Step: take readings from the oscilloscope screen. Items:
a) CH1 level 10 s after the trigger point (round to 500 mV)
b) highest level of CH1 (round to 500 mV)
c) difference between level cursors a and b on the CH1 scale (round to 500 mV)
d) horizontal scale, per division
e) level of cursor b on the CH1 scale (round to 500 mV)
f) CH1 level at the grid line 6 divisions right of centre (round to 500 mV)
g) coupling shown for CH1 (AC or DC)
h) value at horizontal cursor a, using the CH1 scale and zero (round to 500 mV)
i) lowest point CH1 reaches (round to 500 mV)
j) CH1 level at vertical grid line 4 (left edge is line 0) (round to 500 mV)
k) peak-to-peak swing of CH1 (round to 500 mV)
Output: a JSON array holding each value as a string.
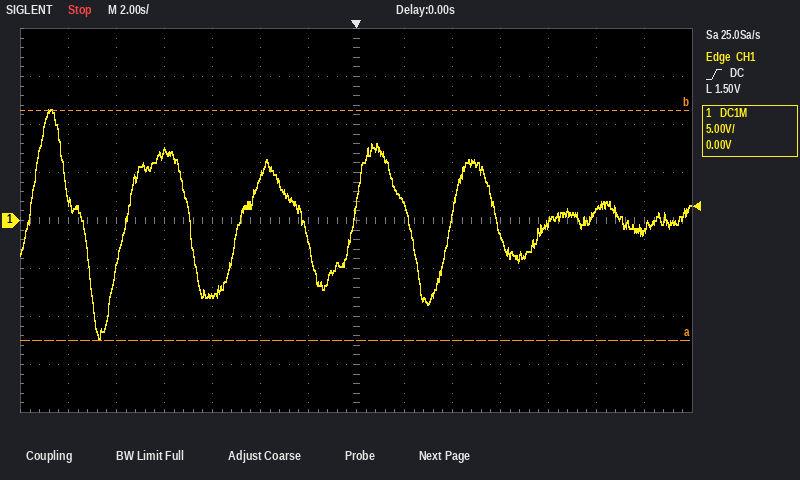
["1.0 V", "11.5 V", "24.0 V", "2 s", "11.5 V", "-1.0 V", "DC", "-12.5 V", "-12.5 V", "-8.0 V", "24.0 V"]
